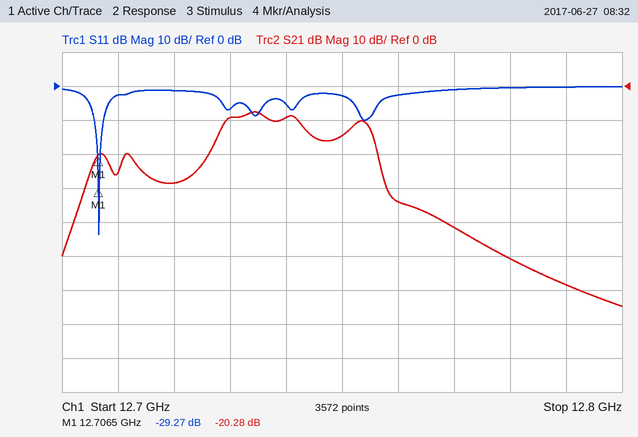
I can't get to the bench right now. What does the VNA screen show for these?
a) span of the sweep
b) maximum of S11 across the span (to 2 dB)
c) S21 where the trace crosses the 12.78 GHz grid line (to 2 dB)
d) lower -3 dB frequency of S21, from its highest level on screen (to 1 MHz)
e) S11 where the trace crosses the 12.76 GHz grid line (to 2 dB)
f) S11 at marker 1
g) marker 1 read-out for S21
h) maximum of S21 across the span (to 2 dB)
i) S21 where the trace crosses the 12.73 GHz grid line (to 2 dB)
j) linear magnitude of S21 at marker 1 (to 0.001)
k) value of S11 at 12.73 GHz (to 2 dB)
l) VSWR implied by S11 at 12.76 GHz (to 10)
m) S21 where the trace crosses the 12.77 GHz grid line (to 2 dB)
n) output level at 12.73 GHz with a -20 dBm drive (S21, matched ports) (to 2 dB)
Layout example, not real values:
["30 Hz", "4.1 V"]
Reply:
["100 MHz", "0 dB", "-50 dB", "12.729 GHz", "-2 dB", "-29.27 dB", "-20.28 dB", "-8 dB", "-10 dB", "0.097", "-6 dB", "10", "-42 dB", "-30 dBm"]
